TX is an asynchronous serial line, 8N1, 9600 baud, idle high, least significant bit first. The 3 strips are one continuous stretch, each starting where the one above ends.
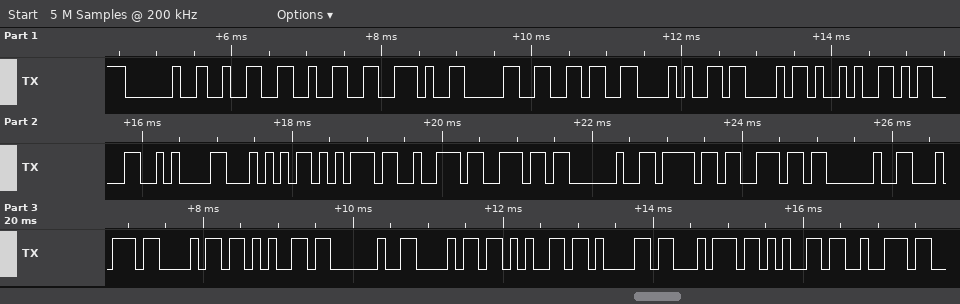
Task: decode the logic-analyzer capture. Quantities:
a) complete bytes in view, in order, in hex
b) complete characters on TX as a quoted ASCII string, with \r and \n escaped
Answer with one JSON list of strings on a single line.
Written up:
["20 32 32 2E 30 36 28 43 29 0D 0A 54 75 72 6E 20 6F 6E 20 74 68 65 20 68 65 61 74 65 72", "\" 22.06(C)\\r\\nTurn on the heater\""]
